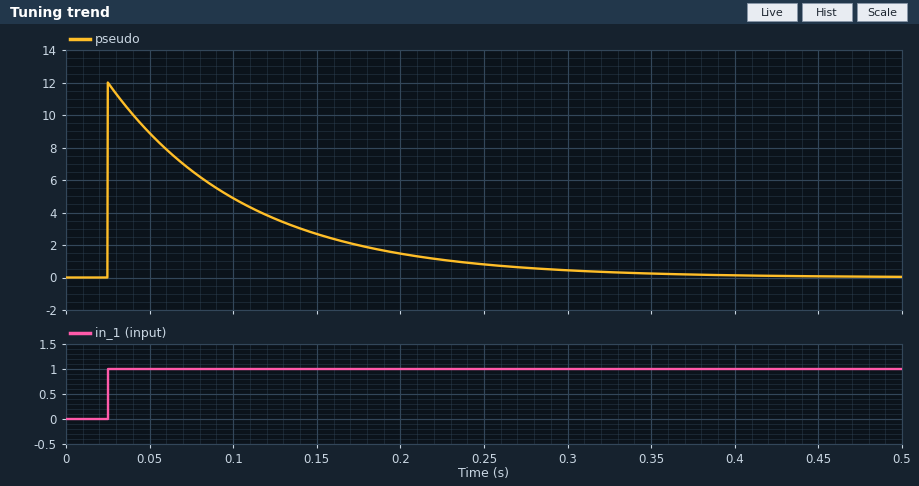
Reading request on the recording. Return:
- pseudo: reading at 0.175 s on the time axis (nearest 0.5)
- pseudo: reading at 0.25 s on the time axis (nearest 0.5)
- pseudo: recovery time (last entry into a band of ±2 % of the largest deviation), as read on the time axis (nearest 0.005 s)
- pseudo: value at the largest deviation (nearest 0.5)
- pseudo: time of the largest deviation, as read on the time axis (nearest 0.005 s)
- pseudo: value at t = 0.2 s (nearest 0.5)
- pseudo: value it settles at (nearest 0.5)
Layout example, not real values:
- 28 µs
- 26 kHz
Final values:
- 2.0
- 1.0
- 0.350 s
- 12.0
- 0.025 s
- 1.5
- 0.0
